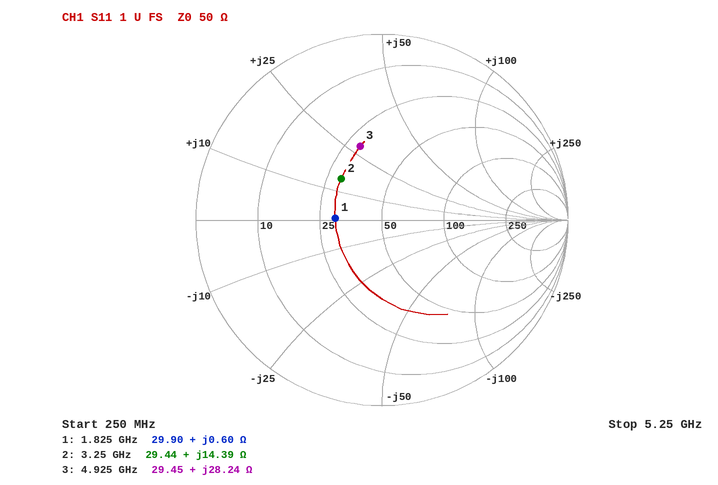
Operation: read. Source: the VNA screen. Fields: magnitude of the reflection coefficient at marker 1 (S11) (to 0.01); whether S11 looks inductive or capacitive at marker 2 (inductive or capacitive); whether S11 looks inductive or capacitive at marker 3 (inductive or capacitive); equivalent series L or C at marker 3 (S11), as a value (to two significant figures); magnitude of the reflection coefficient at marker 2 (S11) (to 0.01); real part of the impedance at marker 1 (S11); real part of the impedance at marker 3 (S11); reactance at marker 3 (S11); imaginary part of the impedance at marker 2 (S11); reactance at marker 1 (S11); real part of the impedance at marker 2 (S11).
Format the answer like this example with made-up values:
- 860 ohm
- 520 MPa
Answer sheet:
- 0.25
- inductive
- inductive
- 910 pH
- 0.31
- 29.90 Ω
- 29.45 Ω
- +28.24 Ω
- +14.39 Ω
- +0.60 Ω
- 29.44 Ω
